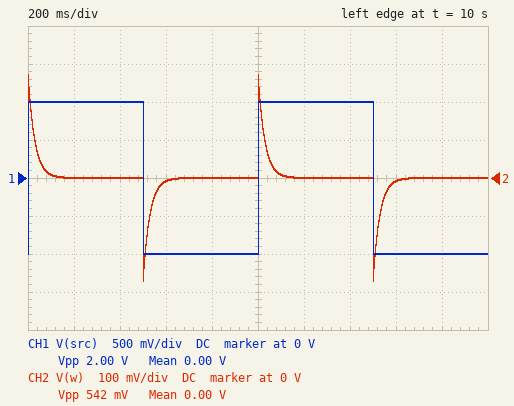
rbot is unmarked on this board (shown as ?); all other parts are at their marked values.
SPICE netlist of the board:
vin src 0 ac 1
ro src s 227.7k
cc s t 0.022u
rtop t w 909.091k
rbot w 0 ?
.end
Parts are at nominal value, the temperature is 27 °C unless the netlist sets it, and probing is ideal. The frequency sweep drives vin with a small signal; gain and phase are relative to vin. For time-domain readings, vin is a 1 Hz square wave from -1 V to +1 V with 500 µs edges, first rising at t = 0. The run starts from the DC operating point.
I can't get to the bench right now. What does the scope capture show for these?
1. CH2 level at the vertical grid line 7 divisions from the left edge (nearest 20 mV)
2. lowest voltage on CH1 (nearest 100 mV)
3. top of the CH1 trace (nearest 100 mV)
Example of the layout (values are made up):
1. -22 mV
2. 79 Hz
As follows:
1. 0 V
2. -1.0 V
3. 1.0 V
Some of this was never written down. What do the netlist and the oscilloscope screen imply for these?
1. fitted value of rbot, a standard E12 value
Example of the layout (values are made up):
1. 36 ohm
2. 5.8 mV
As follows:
1. 180 kΩ
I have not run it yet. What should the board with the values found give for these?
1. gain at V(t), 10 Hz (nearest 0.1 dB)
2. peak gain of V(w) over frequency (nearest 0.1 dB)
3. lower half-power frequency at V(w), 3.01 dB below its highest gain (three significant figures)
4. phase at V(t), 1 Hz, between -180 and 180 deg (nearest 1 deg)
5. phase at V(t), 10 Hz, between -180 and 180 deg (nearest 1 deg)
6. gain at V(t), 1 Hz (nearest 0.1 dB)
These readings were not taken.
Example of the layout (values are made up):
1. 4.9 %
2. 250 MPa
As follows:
1. -2.8 dB
2. -17.3 dB
3. 5.49 Hz
4. 80 deg
5. 29 deg
6. -16.6 dB
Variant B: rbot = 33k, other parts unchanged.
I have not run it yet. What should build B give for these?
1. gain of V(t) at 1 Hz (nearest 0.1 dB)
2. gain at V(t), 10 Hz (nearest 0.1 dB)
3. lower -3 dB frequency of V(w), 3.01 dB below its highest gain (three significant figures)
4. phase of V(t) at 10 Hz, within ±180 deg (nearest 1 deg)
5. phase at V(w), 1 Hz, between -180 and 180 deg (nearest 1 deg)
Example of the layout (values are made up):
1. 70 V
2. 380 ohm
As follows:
1. -17.8 dB
2. -3.3 dB
3. 6.18 Hz
4. 32 deg
5. 81 deg
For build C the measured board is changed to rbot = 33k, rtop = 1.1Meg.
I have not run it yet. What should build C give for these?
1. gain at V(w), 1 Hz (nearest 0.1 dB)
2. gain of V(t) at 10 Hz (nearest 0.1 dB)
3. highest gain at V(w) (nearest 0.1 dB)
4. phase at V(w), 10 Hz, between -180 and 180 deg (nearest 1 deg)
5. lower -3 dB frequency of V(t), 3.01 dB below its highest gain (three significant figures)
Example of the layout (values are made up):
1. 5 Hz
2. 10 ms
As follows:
1. -47.0 dB
2. -2.7 dB
3. -32.3 dB
4. 28 deg
5. 5.32 Hz
